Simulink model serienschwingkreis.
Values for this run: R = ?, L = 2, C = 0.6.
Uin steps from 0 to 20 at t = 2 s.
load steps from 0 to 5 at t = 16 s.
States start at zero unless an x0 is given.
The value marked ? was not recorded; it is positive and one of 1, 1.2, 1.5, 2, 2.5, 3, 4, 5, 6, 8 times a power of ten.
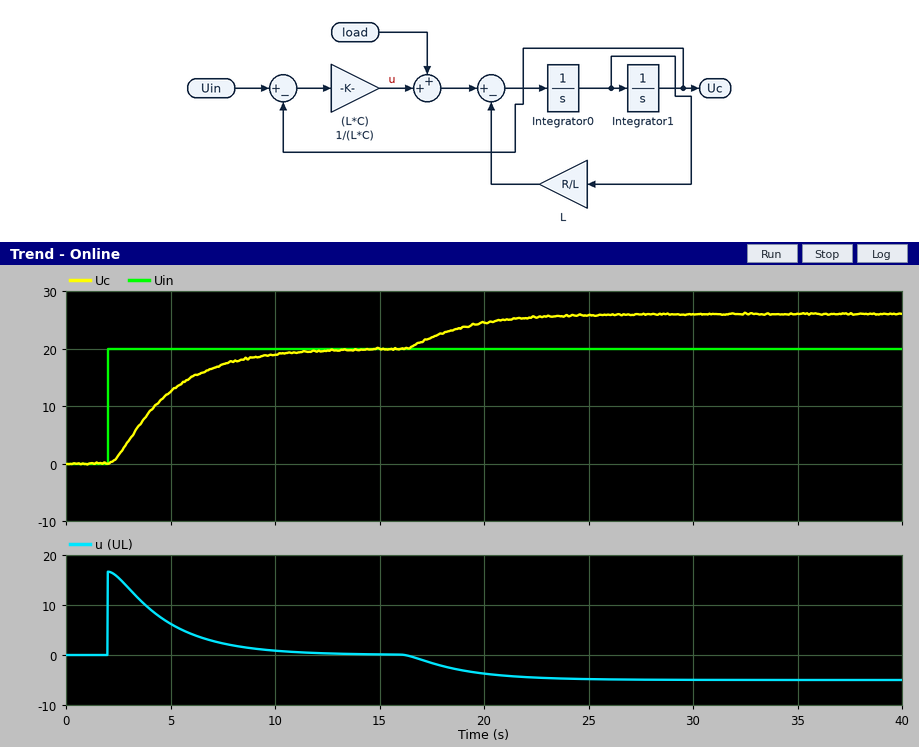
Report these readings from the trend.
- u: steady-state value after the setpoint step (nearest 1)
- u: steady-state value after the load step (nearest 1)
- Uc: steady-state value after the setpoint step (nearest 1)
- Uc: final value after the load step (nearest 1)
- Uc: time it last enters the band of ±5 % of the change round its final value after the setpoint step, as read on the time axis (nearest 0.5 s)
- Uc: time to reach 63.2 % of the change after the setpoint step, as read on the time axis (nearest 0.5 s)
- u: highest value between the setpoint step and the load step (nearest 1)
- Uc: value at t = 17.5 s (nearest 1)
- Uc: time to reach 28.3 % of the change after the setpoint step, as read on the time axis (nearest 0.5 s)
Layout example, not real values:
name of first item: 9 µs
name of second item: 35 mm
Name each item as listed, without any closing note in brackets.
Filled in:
u: steady-state value after the setpoint step: 0
u: steady-state value after the load step: -5
Uc: steady-state value after the setpoint step: 20
Uc: final value after the load step: 26
Uc: time it last enters the band of ±5 % of the change round its final value after the setpoint step, as read on the time axis: 10.0 s
Uc: time to reach 63.2 % of the change after the setpoint step, as read on the time axis: 5.0 s
u: highest value between the setpoint step and the load step: 17
Uc: value at t = 17.5 s: 22
Uc: time to reach 28.3 % of the change after the setpoint step, as read on the time axis: 3.5 s
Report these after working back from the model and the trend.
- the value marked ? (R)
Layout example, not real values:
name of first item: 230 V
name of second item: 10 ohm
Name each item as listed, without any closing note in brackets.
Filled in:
the value marked ?: 5
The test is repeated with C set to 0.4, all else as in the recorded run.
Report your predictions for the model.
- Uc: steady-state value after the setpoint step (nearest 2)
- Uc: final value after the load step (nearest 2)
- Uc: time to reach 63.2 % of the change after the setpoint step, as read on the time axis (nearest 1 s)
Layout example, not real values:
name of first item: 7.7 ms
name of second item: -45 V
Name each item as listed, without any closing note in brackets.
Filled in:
Uc: steady-state value after the setpoint step: 20
Uc: final value after the load step: 24
Uc: time to reach 63.2 % of the change after the setpoint step, as read on the time axis: 4 s
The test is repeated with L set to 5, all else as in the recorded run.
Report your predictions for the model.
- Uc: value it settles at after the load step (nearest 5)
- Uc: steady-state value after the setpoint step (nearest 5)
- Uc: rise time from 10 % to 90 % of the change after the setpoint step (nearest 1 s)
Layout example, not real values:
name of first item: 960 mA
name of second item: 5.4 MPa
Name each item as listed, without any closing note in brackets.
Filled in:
Uc: value it settles at after the load step: 35
Uc: steady-state value after the setpoint step: 20
Uc: rise time from 10 % to 90 % of the change after the setpoint step: 5 s
